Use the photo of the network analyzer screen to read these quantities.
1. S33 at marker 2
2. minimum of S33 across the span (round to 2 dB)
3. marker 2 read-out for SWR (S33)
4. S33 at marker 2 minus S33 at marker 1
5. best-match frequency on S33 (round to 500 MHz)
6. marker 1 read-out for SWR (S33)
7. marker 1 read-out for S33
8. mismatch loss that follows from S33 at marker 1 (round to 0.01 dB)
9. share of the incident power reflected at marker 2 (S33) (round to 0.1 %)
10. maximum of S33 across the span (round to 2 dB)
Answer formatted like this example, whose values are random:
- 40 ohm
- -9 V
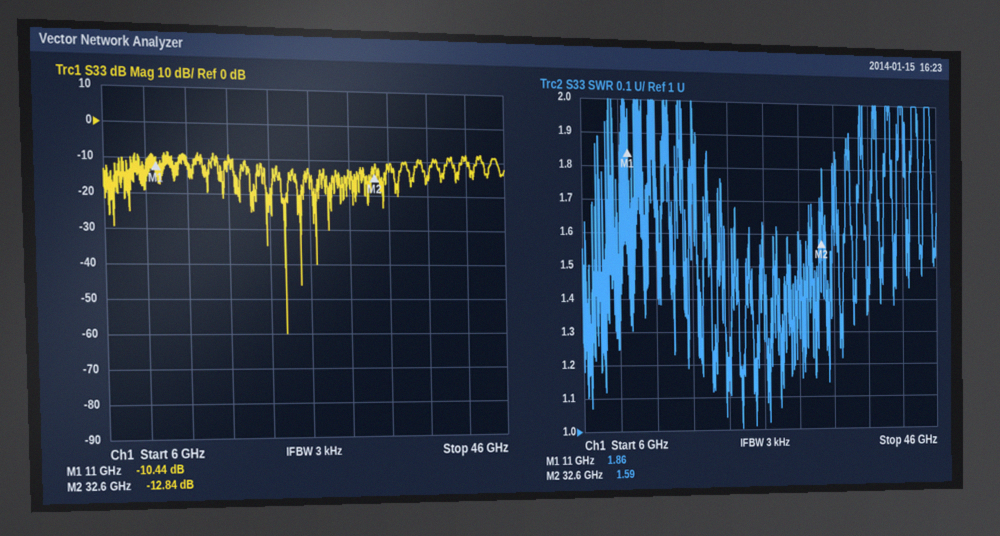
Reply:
- -12.84 dB
- -60 dB
- 1.59
- -2.40 dB
- 23.5 GHz
- 1.86
- -10.44 dB
- 0.41 dB
- 5.2 %
- -8 dB
